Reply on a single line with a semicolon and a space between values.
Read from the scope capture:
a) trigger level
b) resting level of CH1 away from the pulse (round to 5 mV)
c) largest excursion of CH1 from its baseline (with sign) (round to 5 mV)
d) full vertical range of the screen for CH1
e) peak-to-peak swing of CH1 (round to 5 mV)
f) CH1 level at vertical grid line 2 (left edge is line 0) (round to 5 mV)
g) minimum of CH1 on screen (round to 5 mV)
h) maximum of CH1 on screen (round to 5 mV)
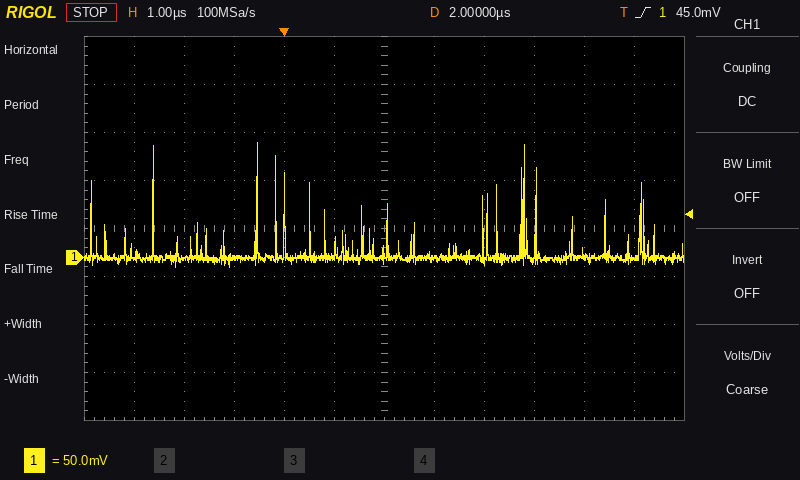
45.0 mV; 0 mV; +120 mV; 400 mV; 130 mV; 0 mV; -10 mV; 120 mV
